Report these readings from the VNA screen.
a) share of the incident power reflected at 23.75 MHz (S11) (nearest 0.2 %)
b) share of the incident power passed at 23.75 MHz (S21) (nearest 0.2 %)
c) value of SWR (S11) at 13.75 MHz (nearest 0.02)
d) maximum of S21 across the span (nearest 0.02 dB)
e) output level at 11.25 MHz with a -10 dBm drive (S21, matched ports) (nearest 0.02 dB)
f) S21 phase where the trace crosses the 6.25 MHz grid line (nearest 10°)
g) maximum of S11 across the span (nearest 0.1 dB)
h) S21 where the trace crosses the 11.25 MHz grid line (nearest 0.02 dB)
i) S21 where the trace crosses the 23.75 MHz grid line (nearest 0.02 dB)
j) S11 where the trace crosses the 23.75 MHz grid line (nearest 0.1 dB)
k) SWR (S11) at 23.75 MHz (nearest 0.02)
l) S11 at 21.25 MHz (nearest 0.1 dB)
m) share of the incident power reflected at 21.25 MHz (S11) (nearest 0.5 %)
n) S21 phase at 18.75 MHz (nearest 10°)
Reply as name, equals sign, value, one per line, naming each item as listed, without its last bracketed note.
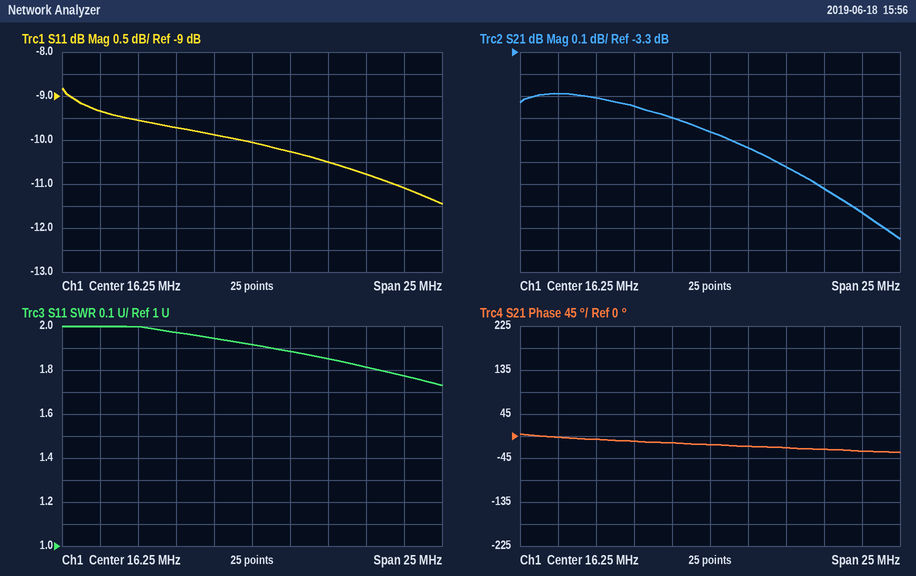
share of the incident power reflected at 23.75 MHz (S11) = 8.4 %
share of the incident power passed at 23.75 MHz (S21) = 40.6 %
value of SWR (S11) at 13.75 MHz = 1.94
maximum of S21 across the span = -3.48 dB
output level at 11.25 MHz with a -10 dBm drive (S21, matched ports) = -13.54 dBm
S21 phase where the trace crosses the 6.25 MHz grid line = 0°
maximum of S11 across the span = -8.8 dB
S21 where the trace crosses the 11.25 MHz grid line = -3.54 dB
S21 where the trace crosses the 23.75 MHz grid line = -3.92 dB
S11 where the trace crosses the 23.75 MHz grid line = -10.8 dB
SWR (S11) at 23.75 MHz = 1.82
S11 at 21.25 MHz = -10.5 dB
share of the incident power reflected at 21.25 MHz (S11) = 9.0 %
S21 phase at 18.75 MHz = -20°
